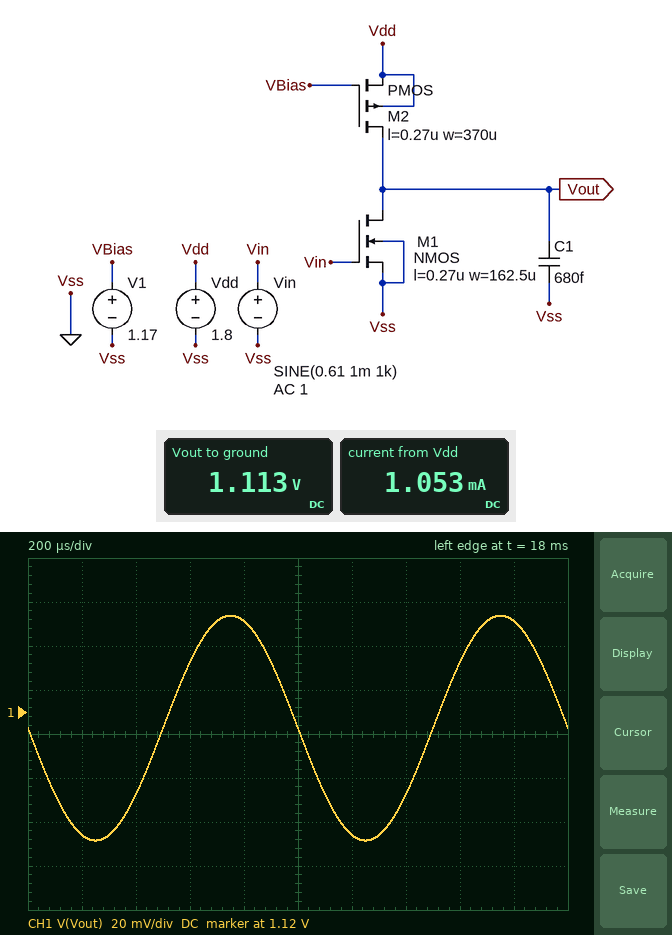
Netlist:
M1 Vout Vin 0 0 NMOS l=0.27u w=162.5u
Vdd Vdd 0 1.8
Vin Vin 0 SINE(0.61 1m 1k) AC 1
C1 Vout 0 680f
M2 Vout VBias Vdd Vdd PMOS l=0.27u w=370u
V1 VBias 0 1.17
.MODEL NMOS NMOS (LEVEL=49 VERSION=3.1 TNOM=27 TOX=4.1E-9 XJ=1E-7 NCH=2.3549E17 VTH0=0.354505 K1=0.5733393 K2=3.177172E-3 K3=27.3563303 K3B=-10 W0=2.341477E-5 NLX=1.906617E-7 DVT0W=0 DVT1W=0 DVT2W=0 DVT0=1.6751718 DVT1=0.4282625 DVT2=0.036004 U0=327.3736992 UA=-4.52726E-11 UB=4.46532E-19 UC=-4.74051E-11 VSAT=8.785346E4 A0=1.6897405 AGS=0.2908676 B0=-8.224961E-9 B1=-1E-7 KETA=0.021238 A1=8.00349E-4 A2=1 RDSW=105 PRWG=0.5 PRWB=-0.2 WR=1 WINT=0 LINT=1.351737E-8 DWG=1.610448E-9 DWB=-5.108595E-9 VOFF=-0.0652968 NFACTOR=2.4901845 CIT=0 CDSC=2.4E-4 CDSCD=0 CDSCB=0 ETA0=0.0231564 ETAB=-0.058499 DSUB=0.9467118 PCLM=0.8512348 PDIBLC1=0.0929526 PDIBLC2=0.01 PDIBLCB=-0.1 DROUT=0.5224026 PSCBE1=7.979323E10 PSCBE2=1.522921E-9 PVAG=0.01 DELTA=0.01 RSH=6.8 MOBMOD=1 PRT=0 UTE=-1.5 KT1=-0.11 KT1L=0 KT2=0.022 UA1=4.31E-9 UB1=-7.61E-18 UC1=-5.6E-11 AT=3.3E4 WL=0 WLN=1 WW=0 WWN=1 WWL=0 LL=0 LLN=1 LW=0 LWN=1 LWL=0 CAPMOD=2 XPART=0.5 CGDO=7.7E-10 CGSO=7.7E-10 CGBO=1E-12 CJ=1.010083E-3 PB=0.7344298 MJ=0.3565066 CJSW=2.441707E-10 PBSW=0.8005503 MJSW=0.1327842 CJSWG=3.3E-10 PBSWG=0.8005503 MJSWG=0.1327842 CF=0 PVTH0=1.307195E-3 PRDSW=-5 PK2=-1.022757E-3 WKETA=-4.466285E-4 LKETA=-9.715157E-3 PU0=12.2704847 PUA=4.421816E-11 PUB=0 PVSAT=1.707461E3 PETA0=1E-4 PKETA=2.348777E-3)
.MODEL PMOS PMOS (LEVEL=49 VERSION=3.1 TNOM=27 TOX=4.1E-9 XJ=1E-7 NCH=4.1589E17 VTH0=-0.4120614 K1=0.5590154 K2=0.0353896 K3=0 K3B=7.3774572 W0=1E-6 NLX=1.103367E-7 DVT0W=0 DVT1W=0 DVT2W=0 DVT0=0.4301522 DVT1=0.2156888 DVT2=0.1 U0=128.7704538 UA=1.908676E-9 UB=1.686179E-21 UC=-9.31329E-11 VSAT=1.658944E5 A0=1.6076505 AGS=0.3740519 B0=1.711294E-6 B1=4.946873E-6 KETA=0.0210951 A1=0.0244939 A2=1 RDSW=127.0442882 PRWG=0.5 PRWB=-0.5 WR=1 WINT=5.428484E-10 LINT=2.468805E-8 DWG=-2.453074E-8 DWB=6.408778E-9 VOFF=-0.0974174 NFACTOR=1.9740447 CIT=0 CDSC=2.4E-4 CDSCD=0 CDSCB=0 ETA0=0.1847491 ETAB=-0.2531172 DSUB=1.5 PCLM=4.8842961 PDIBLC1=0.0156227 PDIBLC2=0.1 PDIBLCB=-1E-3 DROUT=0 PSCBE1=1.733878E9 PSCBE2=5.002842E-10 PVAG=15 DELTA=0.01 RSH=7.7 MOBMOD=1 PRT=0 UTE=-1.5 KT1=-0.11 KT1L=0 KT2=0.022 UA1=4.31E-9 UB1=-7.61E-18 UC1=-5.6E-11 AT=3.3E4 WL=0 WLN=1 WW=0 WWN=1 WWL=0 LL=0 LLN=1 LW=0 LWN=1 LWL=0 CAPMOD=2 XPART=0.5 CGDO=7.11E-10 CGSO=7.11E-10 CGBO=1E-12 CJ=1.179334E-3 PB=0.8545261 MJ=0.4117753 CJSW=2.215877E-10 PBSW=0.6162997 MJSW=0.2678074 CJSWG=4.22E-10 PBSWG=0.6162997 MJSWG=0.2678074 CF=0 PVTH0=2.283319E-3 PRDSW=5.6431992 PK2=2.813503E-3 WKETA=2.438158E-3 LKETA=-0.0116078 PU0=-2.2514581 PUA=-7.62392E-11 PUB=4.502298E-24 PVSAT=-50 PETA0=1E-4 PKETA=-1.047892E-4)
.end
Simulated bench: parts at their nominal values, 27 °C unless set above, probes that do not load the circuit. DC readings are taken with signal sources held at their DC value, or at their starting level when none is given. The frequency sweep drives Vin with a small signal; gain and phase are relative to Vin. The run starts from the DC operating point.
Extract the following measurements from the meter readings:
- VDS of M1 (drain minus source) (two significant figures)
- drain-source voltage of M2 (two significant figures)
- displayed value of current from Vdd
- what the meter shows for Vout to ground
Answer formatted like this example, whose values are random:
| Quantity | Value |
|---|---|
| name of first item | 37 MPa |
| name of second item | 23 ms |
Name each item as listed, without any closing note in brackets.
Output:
| Quantity | Value |
|---|---|
| VDS of M1 (drain minus source) | 1.1 V |
| drain-source voltage of M2 | -690 mV |
| displayed value of current from Vdd | 1.053 mA |
| what the meter shows for Vout to ground | 1.113 V |
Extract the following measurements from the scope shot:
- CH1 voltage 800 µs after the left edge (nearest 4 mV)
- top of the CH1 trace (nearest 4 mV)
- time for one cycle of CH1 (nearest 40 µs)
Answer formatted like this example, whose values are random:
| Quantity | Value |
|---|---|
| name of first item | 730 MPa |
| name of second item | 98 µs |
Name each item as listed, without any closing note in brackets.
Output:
| Quantity | Value |
|---|---|
| CH1 voltage 800 µs after the left edge | 1.160 V |
| top of the CH1 trace | 1.164 V |
| time for one cycle of CH1 | 1.00 ms |
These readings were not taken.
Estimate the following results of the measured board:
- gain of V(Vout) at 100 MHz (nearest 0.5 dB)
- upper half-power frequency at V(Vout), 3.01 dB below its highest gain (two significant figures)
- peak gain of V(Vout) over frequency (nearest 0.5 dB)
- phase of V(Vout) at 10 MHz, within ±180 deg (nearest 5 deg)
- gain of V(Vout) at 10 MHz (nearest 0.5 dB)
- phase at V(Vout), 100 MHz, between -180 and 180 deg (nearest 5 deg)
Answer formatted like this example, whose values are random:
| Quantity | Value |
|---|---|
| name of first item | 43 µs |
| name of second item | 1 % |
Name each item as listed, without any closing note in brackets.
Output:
| Quantity | Value |
|---|---|
| gain of V(Vout) at 100 MHz | 25.0 dB |
| upper half-power frequency at V(Vout), 3.01 dB below its highest gain | 37 MHz |
| peak gain of V(Vout) over frequency | 34.0 dB |
| phase of V(Vout) at 10 MHz, within ±180 deg | 165 deg |
| gain of V(Vout) at 10 MHz | 34.0 dB |
| phase at V(Vout), 100 MHz, between -180 and 180 deg | 110 deg |
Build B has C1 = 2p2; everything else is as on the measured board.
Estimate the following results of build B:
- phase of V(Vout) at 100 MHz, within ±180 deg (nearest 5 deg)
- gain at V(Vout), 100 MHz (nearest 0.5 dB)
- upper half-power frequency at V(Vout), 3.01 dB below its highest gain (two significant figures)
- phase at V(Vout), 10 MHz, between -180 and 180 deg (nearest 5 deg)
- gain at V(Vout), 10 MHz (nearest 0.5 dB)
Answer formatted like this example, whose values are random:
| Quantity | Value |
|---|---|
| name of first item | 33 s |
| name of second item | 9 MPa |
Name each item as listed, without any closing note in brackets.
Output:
| Quantity | Value |
|---|---|
| phase of V(Vout) at 100 MHz, within ±180 deg | 100 deg |
| gain at V(Vout), 100 MHz | 18.5 dB |
| upper half-power frequency at V(Vout), 3.01 dB below its highest gain | 17 MHz |
| phase at V(Vout), 10 MHz, between -180 and 180 deg | 150 deg |
| gain at V(Vout), 10 MHz | 33.0 dB |
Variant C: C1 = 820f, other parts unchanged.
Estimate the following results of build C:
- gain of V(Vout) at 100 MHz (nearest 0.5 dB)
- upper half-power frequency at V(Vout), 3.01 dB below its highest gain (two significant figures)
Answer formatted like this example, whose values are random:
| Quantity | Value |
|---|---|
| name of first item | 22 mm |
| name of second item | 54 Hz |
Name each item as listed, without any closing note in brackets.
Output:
| Quantity | Value |
|---|---|
| gain of V(Vout) at 100 MHz | 24.0 dB |
| upper half-power frequency at V(Vout), 3.01 dB below its highest gain | 33 MHz |
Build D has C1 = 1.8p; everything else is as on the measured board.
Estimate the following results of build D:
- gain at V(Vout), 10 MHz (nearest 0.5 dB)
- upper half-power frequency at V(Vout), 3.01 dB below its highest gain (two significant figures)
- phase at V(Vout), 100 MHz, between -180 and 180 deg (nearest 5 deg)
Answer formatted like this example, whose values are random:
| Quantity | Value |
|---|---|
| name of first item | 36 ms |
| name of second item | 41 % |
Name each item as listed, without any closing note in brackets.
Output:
| Quantity | Value |
|---|---|
| gain at V(Vout), 10 MHz | 33.0 dB |
| upper half-power frequency at V(Vout), 3.01 dB below its highest gain | 19 MHz |
| phase at V(Vout), 100 MHz, between -180 and 180 deg | 100 deg |
